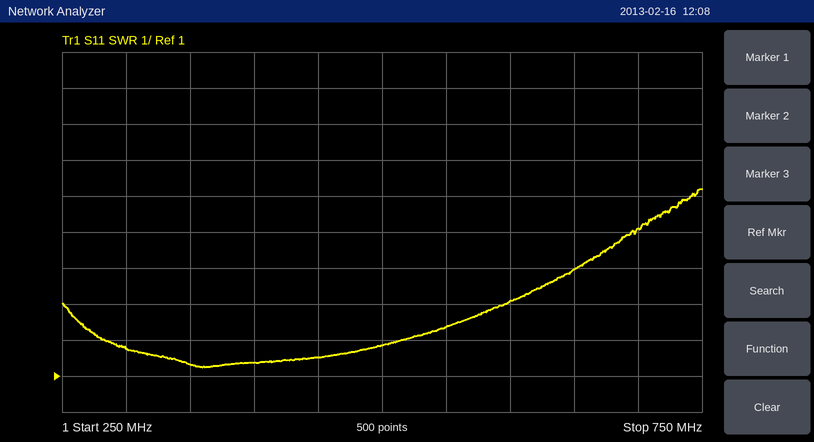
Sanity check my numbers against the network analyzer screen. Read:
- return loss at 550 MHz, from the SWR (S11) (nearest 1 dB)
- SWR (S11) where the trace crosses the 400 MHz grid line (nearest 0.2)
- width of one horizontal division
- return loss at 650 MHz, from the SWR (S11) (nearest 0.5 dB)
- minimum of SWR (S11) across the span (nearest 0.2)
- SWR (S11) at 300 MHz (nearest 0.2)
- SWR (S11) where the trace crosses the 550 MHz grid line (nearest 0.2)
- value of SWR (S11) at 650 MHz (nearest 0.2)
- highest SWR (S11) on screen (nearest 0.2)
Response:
8 dB
1.4
50 MHz
4.5 dB
1.2
1.8
2.4
4.0
6.2
